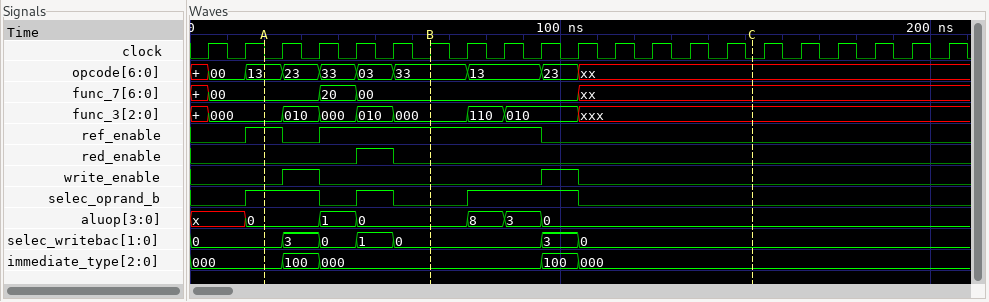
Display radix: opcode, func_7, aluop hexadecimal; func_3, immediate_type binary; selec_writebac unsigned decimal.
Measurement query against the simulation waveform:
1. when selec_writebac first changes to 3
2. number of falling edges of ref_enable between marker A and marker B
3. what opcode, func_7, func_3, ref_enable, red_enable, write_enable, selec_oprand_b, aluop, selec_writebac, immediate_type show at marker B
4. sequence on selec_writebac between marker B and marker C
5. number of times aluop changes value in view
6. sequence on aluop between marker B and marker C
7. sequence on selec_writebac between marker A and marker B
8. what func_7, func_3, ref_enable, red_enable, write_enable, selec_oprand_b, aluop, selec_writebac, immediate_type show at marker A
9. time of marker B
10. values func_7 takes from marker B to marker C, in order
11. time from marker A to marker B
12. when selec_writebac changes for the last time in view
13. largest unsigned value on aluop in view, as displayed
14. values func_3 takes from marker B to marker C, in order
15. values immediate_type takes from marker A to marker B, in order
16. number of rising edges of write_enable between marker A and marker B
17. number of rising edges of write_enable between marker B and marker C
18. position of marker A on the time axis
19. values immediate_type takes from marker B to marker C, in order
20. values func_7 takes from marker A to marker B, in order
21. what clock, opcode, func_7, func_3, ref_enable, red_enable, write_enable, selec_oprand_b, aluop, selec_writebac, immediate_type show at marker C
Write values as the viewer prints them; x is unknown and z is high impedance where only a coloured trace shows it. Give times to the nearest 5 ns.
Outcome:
25 ns
1
opcode=33, func_7=00, func_3=000, ref_enable=1, red_enable=0, write_enable=0, selec_oprand_b=0, aluop=0, selec_writebac=0, immediate_type=000
0, 3, 0
6
0, 8, 3, 0
0, 3, 0, 1, 0
func_7=00, func_3=000, ref_enable=1, red_enable=0, write_enable=0, selec_oprand_b=1, aluop=0, selec_writebac=0, immediate_type=000
65 ns
00, xx
45 ns
105 ns
8
000, 110, 010, xxx
000, 100, 000
1
1
20 ns
000, 100, 000
00, 20, 00
clock=0, opcode=xx, func_7=xx, func_3=xxx, ref_enable=0, red_enable=0, write_enable=0, selec_oprand_b=0, aluop=0, selec_writebac=0, immediate_type=000
